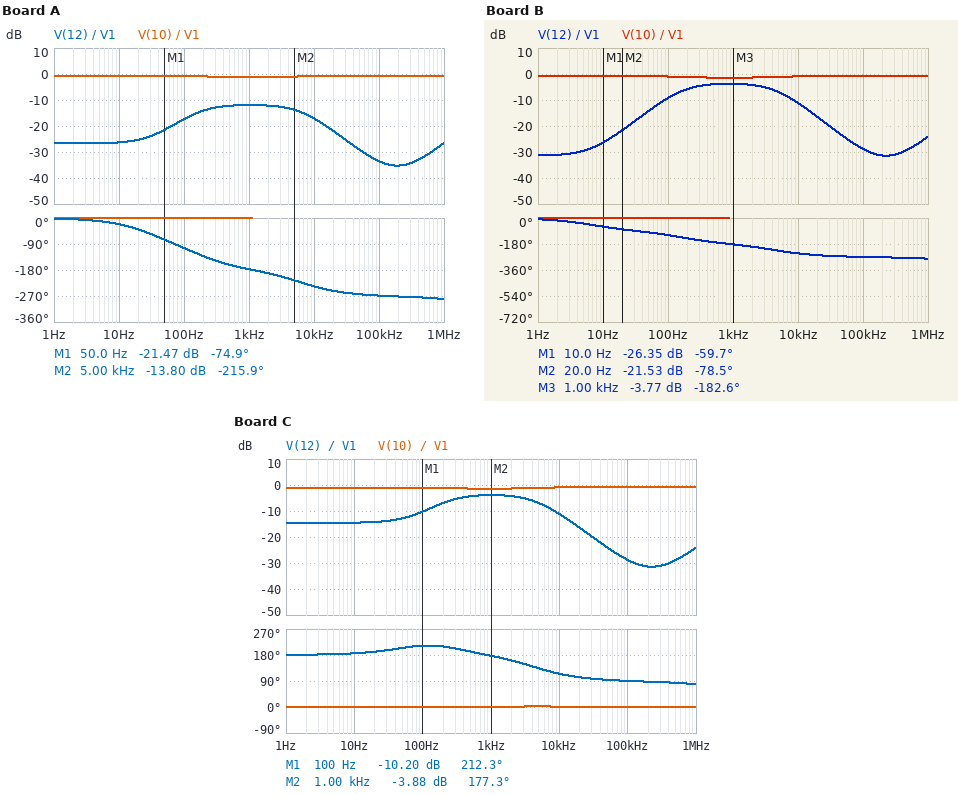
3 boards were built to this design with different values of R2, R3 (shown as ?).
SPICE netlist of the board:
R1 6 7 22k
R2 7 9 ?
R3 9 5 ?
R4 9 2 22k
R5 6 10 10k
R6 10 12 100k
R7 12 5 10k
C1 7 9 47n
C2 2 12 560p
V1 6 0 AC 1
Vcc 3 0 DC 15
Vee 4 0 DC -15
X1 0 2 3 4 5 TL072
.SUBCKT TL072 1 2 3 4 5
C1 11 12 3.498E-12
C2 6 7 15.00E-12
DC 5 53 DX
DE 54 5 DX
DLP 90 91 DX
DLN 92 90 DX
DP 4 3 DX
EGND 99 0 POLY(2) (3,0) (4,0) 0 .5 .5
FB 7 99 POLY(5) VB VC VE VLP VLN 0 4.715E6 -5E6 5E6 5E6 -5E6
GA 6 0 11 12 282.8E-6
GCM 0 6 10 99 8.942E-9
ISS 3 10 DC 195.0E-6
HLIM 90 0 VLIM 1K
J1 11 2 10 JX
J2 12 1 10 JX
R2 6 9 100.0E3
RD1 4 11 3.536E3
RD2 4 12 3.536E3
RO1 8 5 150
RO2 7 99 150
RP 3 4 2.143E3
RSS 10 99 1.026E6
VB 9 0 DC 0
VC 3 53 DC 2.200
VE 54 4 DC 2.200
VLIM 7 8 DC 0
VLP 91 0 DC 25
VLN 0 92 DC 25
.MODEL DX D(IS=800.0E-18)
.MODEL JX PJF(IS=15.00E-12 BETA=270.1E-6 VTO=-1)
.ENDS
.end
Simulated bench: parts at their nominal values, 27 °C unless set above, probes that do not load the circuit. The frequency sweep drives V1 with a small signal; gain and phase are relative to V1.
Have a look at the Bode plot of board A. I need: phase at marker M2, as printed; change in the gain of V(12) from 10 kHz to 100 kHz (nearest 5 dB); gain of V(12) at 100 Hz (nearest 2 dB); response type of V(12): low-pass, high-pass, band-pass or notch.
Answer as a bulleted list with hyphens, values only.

- -215.9 deg
- -15 dB
- -18 dB
- band-pass
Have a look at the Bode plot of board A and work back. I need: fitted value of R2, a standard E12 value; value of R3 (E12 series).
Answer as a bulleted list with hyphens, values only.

- 180 kΩ
- 8.2 kΩ
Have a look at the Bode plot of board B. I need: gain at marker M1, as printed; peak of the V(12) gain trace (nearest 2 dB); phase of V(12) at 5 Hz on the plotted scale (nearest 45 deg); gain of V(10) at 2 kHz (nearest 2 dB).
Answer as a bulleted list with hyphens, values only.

- -26.35 dB
- -4 dB
- -45 deg
- -2 dB
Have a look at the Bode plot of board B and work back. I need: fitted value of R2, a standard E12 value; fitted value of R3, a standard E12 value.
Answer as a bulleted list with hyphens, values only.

- 270 kΩ
- 18 kΩ
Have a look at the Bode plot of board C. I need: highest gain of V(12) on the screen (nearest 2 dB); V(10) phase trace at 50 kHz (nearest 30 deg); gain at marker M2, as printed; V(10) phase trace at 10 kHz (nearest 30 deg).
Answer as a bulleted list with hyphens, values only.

- -4 dB
- 0 deg
- -3.88 dB
- 0 deg
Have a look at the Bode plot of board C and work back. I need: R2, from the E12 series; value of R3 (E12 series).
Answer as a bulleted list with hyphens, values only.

- 39 kΩ
- 18 kΩ
